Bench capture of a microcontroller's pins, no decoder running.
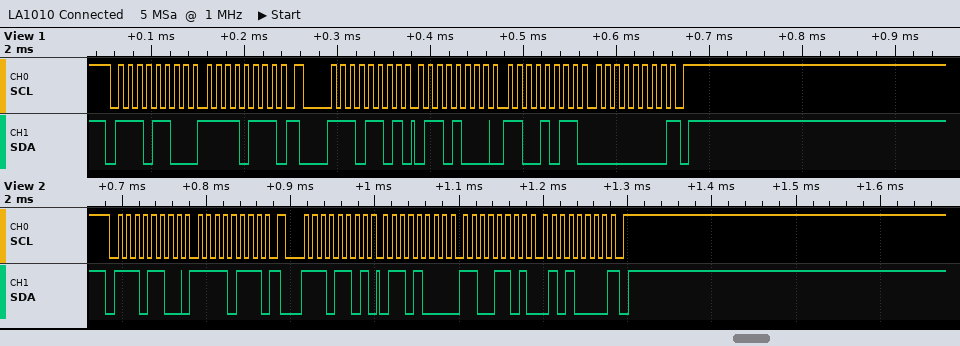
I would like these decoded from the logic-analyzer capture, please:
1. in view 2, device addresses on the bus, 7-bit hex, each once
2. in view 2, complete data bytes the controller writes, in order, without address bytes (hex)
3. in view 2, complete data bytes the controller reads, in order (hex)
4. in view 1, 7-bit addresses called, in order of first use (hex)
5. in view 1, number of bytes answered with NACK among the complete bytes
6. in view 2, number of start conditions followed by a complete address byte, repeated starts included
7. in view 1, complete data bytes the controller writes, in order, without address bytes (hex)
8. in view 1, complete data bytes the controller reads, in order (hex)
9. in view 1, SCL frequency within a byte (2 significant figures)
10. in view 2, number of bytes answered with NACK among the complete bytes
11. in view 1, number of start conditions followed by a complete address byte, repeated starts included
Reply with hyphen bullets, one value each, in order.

- 0x76
- F7
- 68 CD 50
- 0x76
- 1
- 2
- F7
- 68 CB 00
- 100 kHz
- 1
- 2
